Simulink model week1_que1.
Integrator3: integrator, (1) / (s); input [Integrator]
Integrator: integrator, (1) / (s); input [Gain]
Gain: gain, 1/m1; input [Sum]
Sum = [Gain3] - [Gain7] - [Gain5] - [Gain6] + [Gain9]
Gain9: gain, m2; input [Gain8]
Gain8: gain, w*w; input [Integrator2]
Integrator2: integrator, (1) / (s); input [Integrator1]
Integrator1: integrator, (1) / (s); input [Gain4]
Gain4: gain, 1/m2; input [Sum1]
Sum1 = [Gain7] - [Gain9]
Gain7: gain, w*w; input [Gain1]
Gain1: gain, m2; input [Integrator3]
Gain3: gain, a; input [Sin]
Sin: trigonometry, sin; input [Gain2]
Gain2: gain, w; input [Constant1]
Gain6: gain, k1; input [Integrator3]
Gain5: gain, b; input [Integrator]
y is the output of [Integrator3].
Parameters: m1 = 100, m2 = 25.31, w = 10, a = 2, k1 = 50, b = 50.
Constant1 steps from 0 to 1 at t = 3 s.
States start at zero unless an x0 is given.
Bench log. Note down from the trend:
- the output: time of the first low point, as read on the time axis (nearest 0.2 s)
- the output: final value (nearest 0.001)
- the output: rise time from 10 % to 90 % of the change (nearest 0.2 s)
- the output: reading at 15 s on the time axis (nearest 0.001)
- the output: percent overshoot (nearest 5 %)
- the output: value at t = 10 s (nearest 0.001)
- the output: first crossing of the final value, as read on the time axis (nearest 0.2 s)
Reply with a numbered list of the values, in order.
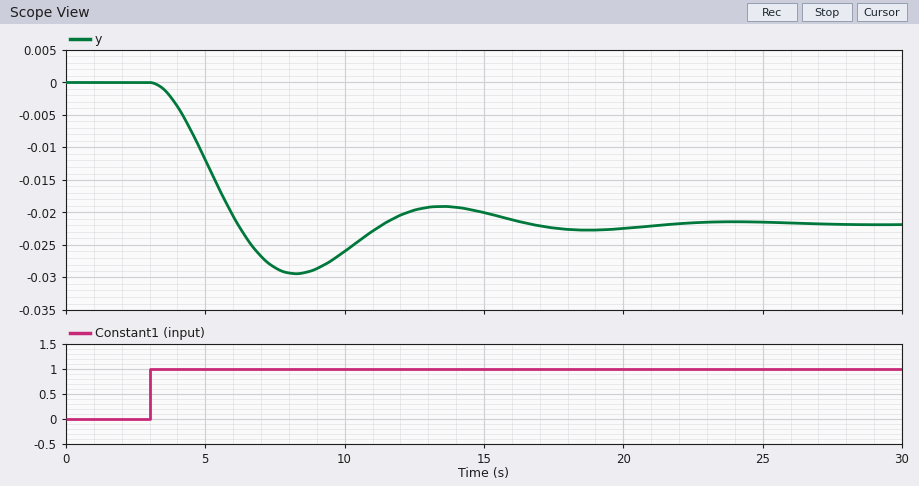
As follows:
1. 8.2 s
2. -0.022
3. 2.2 s
4. -0.020
5. 35 %
6. -0.026
7. 6.2 s
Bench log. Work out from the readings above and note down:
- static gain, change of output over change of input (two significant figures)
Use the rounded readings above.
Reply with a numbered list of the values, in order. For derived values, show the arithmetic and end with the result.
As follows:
1. (-0.022 - 0) / (1 - 0) = -0.022
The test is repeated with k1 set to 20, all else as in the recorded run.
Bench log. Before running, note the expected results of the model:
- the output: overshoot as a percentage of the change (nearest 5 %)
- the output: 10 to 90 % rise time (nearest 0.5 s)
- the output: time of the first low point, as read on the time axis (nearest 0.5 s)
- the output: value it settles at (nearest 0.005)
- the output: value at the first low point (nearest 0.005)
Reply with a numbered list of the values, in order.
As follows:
1. 15 %
2. 4.0 s
3. 12.0 s
4. -0.055
5. -0.065
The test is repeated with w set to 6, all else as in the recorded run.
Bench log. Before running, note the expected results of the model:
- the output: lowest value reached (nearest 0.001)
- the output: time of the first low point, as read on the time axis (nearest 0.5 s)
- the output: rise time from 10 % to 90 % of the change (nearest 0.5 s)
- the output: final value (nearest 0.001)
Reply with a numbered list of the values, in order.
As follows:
1. -0.015
2. 8.0 s
3. 2.0 s
4. -0.011
